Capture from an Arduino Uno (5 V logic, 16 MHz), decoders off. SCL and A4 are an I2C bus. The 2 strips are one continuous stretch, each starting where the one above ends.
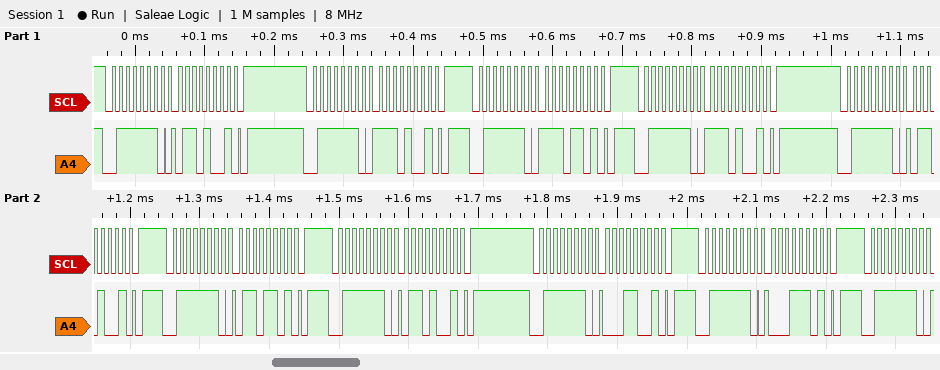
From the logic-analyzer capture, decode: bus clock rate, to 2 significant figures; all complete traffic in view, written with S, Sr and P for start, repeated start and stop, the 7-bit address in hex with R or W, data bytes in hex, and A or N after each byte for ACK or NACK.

100 kHz
S 3FW A 69 A P S 3FW A E9 A P S 3FW A ED A P S 3FW A E9 A P S 3FW A 69 A P S 3FW A 6D A P S 3FW A 69 A P S 3FW A 19 A P S 3FW A 1D A P S 3FW A
